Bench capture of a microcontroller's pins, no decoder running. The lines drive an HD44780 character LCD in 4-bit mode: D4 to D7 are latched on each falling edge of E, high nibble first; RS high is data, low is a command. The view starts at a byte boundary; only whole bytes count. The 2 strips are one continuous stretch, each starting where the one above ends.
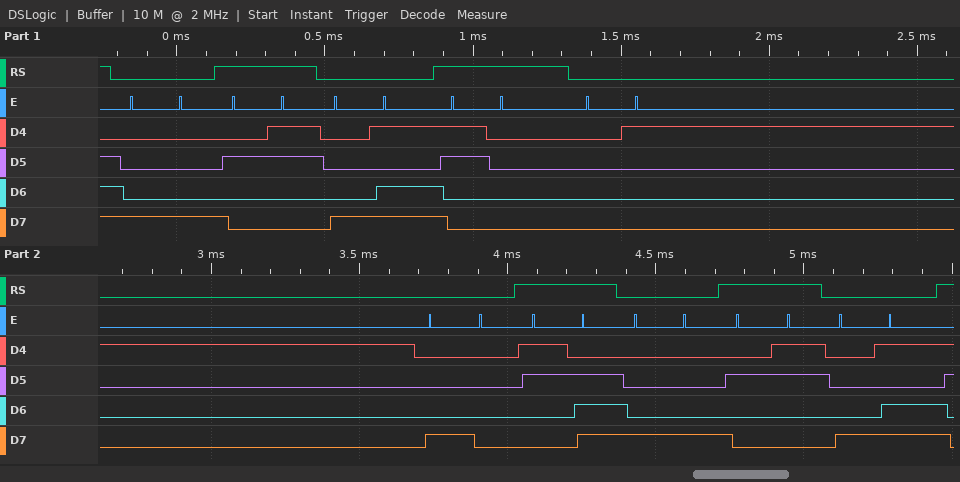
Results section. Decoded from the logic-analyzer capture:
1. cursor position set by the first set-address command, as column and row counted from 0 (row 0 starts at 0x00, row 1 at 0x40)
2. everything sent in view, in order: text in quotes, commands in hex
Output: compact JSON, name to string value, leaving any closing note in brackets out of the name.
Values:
{"cursor position set by the first set-address command, as column and row counted from 0": "column 8, row 0", "everything sent in view, in order: text in quotes, commands in hex": "0x88 \"#\" 0x8D \"0\" 0x01 0x80 \">\" 0x88 \"#\" 0x8D"}
